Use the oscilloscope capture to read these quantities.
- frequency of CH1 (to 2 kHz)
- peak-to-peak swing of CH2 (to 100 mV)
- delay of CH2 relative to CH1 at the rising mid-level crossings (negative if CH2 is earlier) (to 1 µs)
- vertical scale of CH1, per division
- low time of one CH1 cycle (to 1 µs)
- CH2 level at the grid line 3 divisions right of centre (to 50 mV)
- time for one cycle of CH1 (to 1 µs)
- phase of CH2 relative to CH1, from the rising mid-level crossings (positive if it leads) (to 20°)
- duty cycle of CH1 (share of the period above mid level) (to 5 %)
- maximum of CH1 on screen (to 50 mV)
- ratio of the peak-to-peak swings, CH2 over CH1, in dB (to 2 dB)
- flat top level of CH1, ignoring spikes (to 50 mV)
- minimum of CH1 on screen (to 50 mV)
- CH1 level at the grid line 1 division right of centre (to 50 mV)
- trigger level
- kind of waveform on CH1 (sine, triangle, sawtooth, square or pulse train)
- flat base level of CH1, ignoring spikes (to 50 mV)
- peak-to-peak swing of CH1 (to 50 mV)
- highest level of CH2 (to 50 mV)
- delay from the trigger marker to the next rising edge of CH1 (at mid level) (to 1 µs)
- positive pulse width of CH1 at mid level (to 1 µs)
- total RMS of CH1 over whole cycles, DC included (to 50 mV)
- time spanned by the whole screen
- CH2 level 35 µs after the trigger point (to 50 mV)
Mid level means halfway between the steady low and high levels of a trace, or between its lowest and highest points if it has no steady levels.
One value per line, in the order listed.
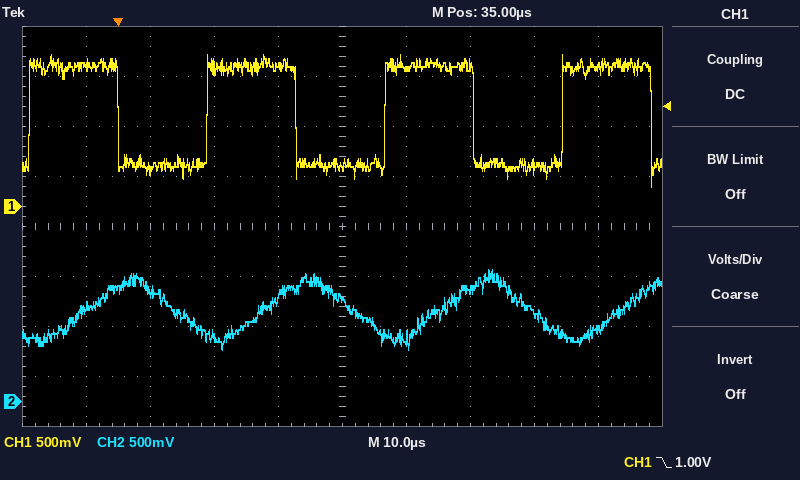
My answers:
36 kHz
800 mV
+9 µs
500 mV
14 µs
900 mV
28 µs
-120°
50 %
1.50 V
-4 dB
1.40 V
200 mV
1.40 V
1.00 V
square
400 mV
1.30 V
1.30 V
14 µs
14 µs
1.05 V
100 µs
1.05 V
